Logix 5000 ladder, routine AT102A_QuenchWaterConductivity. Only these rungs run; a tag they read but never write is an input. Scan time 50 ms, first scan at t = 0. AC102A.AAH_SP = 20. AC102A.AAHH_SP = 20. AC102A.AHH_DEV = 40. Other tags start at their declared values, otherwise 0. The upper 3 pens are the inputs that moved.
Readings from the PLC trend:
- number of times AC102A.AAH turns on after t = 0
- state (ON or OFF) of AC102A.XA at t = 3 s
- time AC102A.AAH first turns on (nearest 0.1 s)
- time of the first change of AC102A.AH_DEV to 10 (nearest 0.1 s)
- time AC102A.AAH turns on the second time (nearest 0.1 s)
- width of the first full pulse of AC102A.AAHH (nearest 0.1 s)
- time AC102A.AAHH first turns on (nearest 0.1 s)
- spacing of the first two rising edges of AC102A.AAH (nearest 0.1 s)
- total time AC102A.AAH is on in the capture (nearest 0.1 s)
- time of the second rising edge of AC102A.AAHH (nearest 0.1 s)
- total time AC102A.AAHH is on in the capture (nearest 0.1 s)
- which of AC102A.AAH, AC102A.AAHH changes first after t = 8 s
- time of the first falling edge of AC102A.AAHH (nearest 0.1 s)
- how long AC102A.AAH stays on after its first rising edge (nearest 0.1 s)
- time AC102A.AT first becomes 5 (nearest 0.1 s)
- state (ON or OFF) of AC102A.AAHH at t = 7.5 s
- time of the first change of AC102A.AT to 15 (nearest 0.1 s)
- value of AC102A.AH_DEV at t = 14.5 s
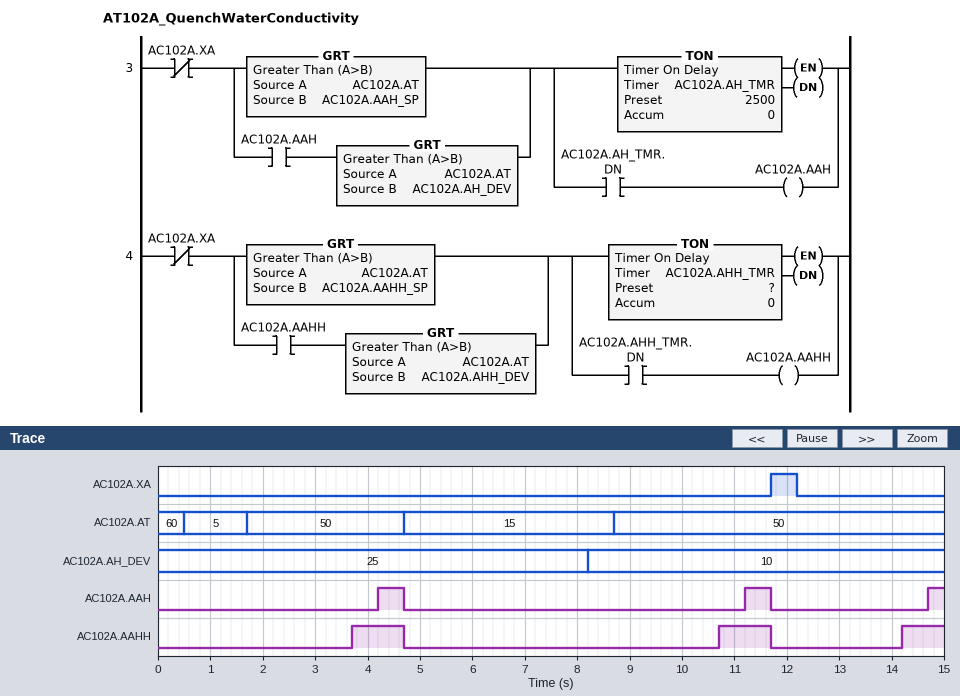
3
OFF
4.2 s
8.2 s
11.2 s
1.0 s
3.7 s
7.0 s
1.3 s
10.7 s
2.8 s
AC102A.AAHH
4.7 s
0.5 s
0.5 s
OFF
4.7 s
10
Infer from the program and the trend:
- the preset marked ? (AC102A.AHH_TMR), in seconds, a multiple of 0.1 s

2.0 s
